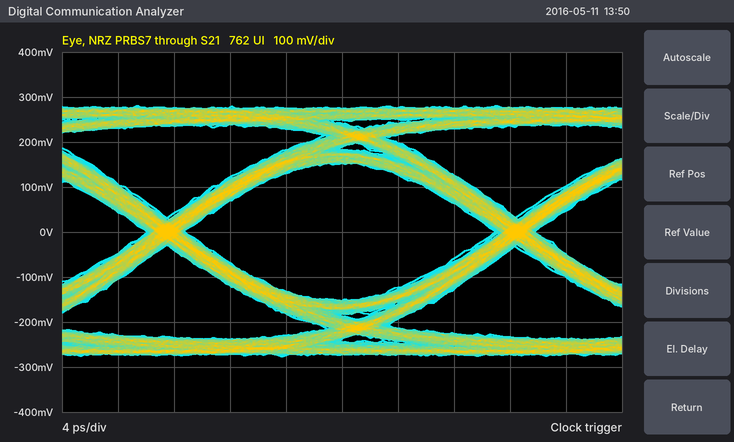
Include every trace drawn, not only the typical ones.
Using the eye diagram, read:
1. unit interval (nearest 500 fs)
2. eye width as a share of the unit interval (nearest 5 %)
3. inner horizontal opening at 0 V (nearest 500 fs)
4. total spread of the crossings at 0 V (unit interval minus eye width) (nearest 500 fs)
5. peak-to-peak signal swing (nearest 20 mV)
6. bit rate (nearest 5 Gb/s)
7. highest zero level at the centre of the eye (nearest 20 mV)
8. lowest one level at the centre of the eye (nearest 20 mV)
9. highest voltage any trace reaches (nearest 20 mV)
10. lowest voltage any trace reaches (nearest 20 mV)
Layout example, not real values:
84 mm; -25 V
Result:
25.0 ps; 90 %; 22.0 ps; 3.0 ps; 560 mV; 40 Gb/s; -160 mV; 160 mV; 280 mV; -280 mV
